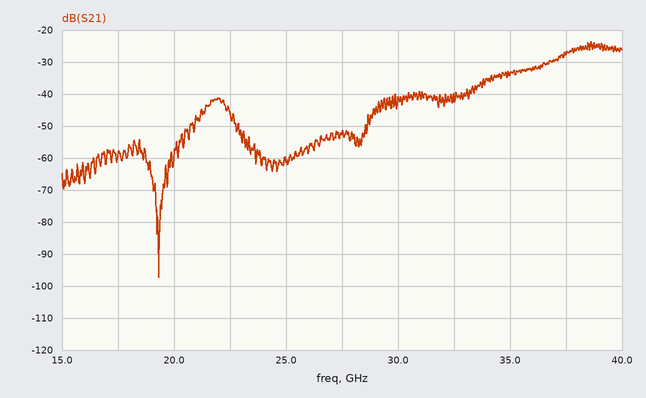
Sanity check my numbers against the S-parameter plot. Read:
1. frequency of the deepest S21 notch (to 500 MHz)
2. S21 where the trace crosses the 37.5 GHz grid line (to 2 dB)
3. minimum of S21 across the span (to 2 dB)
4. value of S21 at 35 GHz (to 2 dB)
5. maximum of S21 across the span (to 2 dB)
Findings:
19.5 GHz
-28 dB
-98 dB
-34 dB
-24 dB
